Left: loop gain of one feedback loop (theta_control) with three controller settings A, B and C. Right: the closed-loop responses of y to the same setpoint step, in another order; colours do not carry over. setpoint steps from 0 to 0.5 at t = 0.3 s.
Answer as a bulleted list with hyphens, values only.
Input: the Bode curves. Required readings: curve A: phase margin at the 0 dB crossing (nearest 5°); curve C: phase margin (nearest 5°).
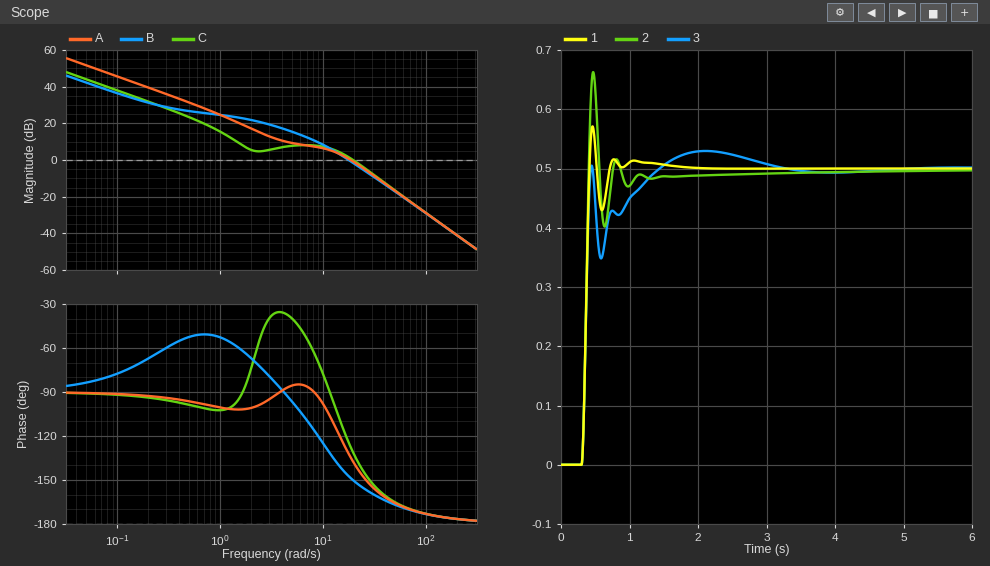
- 45°
- 50°
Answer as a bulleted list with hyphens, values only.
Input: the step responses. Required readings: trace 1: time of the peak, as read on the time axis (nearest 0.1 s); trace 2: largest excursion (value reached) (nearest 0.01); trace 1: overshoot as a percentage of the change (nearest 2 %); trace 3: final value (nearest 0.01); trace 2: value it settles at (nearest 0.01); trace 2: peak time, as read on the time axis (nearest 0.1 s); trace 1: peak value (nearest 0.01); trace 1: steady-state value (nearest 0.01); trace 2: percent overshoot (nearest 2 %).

- 0.5 s
- 0.66
- 14 %
- 0.50
- 0.50
- 0.5 s
- 0.57
- 0.50
- 32 %
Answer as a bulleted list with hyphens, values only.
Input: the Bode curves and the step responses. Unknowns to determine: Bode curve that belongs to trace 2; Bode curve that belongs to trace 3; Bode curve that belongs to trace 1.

- B
- C
- A
